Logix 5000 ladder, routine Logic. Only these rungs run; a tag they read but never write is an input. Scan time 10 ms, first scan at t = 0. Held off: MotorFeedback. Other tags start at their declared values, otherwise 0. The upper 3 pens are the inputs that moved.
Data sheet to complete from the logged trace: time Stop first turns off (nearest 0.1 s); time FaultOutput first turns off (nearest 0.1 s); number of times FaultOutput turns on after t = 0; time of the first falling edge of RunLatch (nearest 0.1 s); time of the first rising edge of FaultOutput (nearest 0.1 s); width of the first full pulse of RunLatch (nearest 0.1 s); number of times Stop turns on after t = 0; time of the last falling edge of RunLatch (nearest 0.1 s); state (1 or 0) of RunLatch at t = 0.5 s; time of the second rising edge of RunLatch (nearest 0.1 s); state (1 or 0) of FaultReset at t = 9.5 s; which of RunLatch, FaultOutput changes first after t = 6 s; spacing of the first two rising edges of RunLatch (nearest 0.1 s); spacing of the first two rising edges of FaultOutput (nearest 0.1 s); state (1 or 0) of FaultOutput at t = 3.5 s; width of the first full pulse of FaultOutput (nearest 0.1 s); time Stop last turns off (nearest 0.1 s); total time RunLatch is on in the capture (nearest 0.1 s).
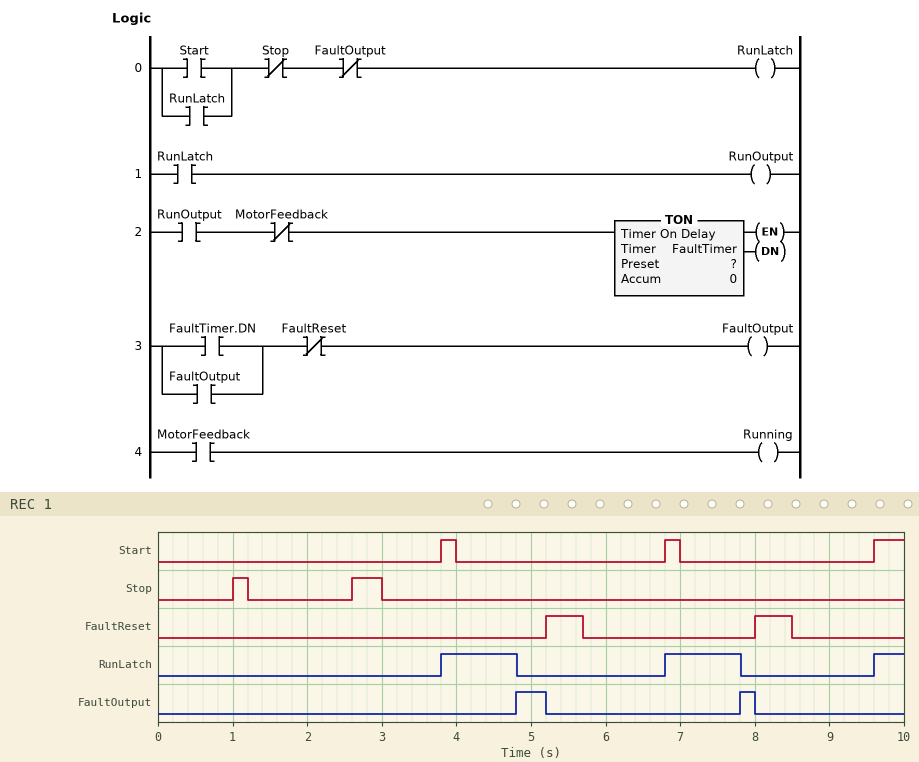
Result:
1.2 s
5.2 s
2
4.8 s
4.8 s
1.0 s
2
7.8 s
0
6.8 s
0
RunLatch
3.0 s
3.0 s
0
0.4 s
3.0 s
2.4 s
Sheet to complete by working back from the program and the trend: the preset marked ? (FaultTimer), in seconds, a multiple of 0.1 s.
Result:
1.0 s
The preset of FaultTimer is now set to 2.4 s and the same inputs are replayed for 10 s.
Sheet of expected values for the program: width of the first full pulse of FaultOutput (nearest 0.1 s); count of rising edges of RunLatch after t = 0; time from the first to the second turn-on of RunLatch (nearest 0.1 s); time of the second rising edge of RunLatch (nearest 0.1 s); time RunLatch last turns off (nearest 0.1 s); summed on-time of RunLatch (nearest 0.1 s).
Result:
1.8 s
2
5.8 s
9.6 s
6.2 s
2.8 s
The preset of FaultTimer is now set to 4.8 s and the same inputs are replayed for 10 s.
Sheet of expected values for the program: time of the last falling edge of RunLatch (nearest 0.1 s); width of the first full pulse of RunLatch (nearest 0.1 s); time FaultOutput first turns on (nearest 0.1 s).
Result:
8.6 s
4.8 s
8.6 s
